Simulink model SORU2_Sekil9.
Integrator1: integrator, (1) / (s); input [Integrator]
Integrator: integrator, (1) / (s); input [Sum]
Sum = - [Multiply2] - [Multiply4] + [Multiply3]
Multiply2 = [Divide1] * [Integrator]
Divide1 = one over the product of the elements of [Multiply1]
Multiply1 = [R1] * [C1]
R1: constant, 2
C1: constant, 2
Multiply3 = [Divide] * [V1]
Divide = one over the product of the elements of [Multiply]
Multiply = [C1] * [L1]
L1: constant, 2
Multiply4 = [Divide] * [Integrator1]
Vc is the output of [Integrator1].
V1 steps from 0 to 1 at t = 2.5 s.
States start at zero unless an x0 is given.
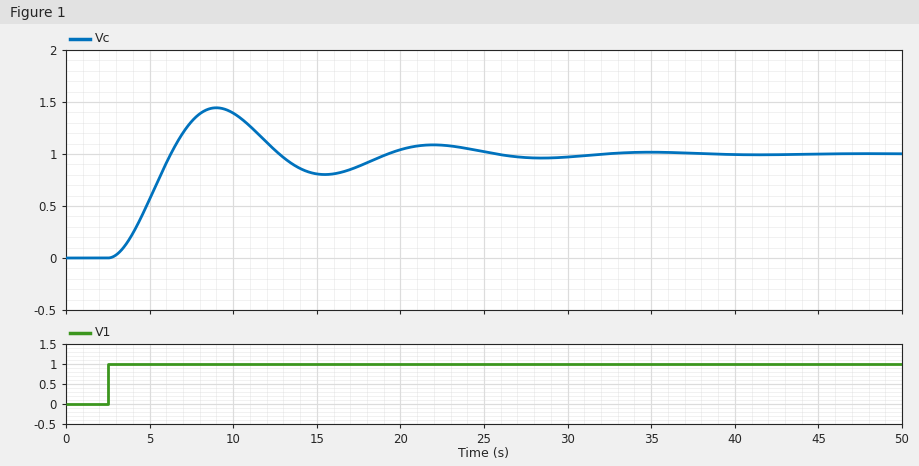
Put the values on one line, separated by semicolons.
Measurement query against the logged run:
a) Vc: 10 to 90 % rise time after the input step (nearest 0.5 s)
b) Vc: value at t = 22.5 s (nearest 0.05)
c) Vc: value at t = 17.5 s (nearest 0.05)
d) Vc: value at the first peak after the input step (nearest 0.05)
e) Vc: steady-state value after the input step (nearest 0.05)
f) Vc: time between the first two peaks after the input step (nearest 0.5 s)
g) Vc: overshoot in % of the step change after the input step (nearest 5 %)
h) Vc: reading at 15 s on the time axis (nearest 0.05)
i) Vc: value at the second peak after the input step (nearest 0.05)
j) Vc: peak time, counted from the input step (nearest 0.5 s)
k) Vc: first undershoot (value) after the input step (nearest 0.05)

2.5 s; 1.10; 0.90; 1.45; 1.00; 13.0 s; 45 %; 0.80; 1.10; 6.5 s; 0.80
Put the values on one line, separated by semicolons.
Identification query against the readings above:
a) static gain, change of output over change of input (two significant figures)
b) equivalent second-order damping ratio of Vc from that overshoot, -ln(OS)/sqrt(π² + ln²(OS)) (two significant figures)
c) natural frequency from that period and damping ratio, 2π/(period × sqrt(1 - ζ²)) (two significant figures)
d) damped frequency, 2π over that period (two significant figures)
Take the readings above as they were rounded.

1.0; 0.25; 0.50 rad/s; 0.48 rad/s
